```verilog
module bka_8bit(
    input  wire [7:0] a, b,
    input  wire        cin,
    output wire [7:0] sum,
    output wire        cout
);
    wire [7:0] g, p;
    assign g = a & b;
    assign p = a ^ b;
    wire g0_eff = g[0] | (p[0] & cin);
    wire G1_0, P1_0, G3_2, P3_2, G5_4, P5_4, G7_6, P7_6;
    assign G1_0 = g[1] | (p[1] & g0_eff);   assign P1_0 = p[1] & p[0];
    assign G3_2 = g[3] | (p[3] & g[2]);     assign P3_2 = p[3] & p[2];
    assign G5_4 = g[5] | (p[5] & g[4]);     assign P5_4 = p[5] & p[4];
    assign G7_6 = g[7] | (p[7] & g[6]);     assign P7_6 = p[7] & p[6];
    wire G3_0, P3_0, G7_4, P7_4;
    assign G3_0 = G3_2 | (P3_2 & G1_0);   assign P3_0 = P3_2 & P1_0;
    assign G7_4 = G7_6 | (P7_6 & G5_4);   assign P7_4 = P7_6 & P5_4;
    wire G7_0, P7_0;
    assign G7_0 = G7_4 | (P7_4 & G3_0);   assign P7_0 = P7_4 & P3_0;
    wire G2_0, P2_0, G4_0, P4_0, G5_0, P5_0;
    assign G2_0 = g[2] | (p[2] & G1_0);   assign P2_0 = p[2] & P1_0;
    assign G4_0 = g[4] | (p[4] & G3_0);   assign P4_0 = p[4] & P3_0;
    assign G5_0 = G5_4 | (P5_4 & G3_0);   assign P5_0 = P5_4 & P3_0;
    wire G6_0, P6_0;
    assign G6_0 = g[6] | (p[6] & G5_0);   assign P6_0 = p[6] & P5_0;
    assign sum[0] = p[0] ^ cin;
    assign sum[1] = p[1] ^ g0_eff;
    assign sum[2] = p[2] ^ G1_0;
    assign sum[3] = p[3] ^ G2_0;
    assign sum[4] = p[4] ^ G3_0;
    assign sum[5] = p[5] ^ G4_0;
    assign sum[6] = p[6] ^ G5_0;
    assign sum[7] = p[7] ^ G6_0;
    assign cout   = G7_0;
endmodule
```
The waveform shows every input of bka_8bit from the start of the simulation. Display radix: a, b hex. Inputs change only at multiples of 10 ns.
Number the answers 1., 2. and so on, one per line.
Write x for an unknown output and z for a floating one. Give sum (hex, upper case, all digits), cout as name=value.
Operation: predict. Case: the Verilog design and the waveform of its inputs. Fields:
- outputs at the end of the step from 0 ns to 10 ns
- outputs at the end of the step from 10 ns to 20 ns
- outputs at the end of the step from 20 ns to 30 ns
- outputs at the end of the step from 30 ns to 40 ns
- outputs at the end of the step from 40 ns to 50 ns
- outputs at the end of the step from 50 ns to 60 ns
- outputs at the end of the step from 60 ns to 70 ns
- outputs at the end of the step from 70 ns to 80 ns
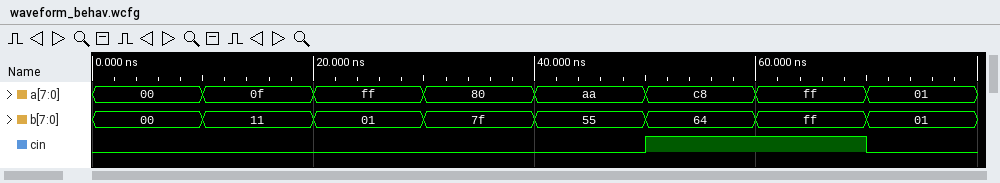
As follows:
1. sum=00, cout=0
2. sum=20, cout=0
3. sum=00, cout=1
4. sum=FF, cout=0
5. sum=FF, cout=0
6. sum=2D, cout=1
7. sum=FF, cout=1
8. sum=02, cout=0
